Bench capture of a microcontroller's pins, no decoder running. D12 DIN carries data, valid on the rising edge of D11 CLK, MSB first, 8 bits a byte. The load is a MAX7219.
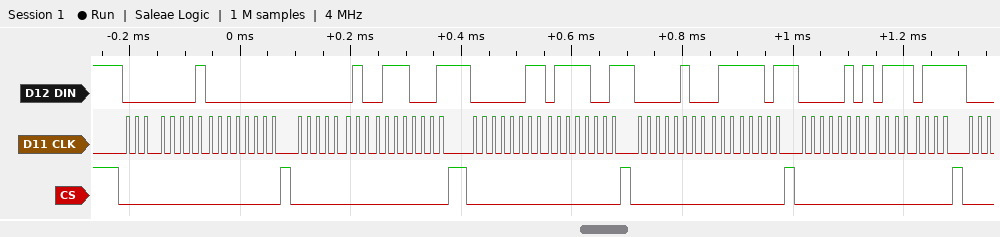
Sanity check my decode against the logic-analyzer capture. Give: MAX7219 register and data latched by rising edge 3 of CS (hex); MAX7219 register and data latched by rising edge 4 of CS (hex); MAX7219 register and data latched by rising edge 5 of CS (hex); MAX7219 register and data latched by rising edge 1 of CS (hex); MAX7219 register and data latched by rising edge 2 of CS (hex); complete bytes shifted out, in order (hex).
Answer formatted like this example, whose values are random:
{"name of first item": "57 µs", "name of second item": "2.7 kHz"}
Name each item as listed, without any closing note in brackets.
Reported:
{"MAX7219 register and data latched by rising edge 3 of CS": "register 0x3, data 0x79", "MAX7219 register and data latched by rising edge 4 of CS": "register 0x4, data 0x7D", "MAX7219 register and data latched by rising edge 5 of CS": "register 0x5, data 0x77", "MAX7219 register and data latched by rising edge 1 of CS": "register 0x1, data 0x00", "MAX7219 register and data latched by rising edge 2 of CS": "register 0x2, data 0x71", "complete bytes shifted out, in order": "01 00 02 71 03 79 04 7D 05 77"}
